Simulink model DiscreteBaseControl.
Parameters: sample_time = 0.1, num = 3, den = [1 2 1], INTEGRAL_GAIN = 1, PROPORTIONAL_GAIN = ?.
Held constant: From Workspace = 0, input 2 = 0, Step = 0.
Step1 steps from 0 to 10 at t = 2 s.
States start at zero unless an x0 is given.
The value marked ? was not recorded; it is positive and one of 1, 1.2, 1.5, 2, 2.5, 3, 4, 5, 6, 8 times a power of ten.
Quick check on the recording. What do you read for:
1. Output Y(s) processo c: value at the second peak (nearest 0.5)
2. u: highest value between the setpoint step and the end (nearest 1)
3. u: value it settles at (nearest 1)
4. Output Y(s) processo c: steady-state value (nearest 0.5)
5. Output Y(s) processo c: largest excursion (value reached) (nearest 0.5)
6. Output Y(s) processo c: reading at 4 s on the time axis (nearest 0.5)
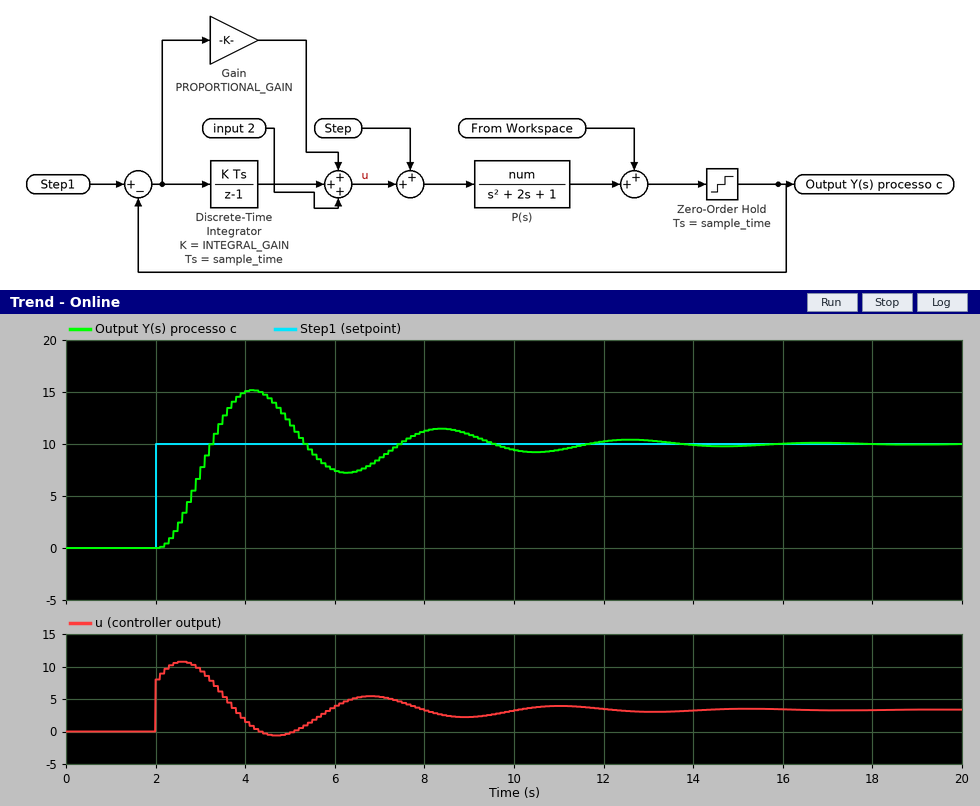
11.5
11
3
10.0
15.0
15.0
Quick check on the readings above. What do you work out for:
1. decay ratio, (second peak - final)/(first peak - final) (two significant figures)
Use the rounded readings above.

0.30
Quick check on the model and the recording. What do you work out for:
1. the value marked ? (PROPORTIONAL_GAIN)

0.8
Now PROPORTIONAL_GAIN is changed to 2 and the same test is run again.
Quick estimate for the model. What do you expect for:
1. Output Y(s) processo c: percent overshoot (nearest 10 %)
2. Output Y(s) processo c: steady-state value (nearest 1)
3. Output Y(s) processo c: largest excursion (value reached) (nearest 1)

40 %
10
14
